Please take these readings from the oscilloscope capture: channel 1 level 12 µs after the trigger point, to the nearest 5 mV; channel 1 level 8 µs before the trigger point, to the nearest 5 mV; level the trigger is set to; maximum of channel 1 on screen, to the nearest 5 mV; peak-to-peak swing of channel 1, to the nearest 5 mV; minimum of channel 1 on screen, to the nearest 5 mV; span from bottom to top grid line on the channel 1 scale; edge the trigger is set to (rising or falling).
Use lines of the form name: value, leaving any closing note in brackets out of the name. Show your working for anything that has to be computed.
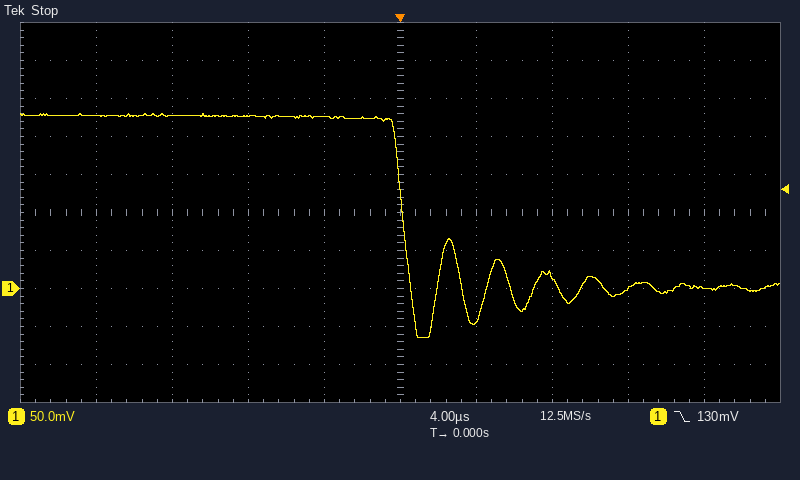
channel 1 level 12 µs after the trigger point, to the nearest 5 mV: 0 mV
channel 1 level 8 µs before the trigger point, to the nearest 5 mV: 225 mV
level the trigger is set to: 130 mV
maximum of channel 1 on screen, to the nearest 5 mV: 230 mV
peak-to-peak swing of channel 1, to the nearest 5 mV: 230 mV − (-65 mV) = 295 mV
minimum of channel 1 on screen, to the nearest 5 mV: -65 mV
span from bottom to top grid line on the channel 1 scale: 500 mV
edge the trigger is set to: falling
